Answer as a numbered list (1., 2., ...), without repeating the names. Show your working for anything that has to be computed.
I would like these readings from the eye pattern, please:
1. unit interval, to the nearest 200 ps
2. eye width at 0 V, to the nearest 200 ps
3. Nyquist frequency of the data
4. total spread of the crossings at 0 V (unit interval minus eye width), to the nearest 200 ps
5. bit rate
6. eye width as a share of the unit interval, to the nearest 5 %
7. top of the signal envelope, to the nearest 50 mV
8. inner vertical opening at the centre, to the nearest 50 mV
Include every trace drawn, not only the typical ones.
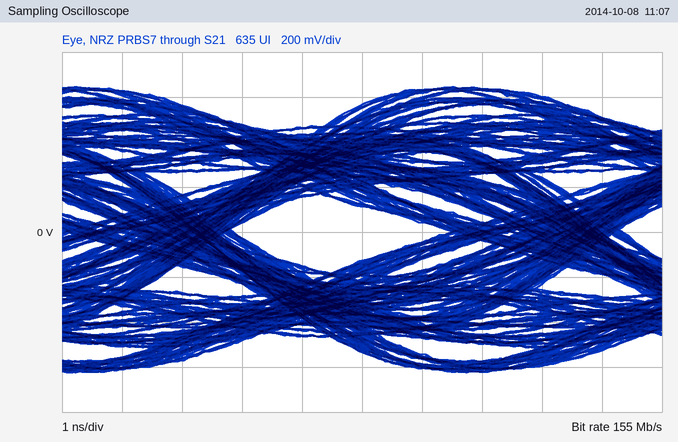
1. 6.4 ns
2. 3.6 ns
3. 77.5 MHz
4. 2.8 ns
5. 155 Mb/s
6. 3.6 ns / 6.4 ns ≈ 56.2 %, so 55 % to the nearest 5 %
7. 650 mV
8. 250 mV
